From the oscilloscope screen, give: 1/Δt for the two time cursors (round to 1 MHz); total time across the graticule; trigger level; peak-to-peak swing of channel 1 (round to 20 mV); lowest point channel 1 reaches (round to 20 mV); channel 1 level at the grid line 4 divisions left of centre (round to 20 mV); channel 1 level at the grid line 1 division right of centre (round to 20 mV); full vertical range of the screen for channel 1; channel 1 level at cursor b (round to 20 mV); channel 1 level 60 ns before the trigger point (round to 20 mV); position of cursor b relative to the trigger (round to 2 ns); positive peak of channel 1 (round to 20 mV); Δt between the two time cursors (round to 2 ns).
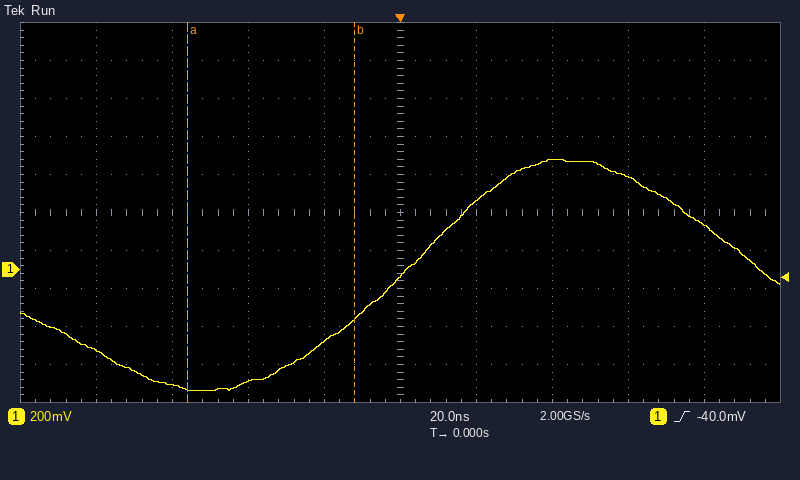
23 MHz
200 ns
-40.0 mV
1.22 V
-640 mV
-420 mV
360 mV
2 V
-260 mV
-600 mV
-12 ns
580 mV
44 ns
